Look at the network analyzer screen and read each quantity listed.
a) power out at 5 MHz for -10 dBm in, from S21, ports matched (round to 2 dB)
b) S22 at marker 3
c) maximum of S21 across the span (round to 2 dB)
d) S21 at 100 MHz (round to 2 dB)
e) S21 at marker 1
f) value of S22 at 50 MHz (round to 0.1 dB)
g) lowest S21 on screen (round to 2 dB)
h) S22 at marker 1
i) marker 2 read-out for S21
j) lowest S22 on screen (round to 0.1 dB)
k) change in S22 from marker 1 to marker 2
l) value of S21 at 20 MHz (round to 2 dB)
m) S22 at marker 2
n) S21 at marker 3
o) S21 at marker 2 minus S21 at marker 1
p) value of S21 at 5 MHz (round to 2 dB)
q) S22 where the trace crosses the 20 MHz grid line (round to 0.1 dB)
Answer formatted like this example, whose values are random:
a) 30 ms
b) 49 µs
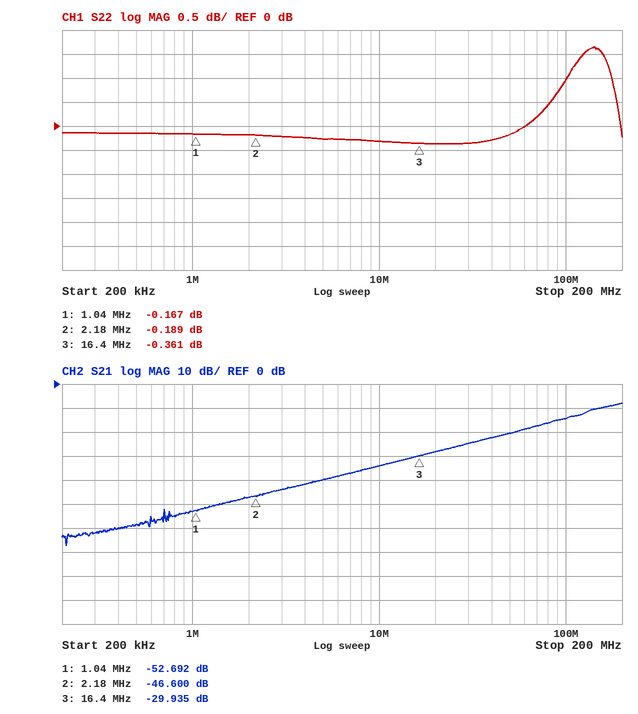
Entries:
a) -50 dBm
b) -0.361 dB
c) -8 dB
d) -14 dB
e) -52.692 dB
f) -0.2 dB
g) -68 dB
h) -0.167 dB
i) -46.600 dB
j) -0.4 dB
k) -0.022 dB
l) -28 dB
m) -0.189 dB
n) -29.935 dB
o) 6.092 dB
p) -40 dB
q) -0.4 dB
